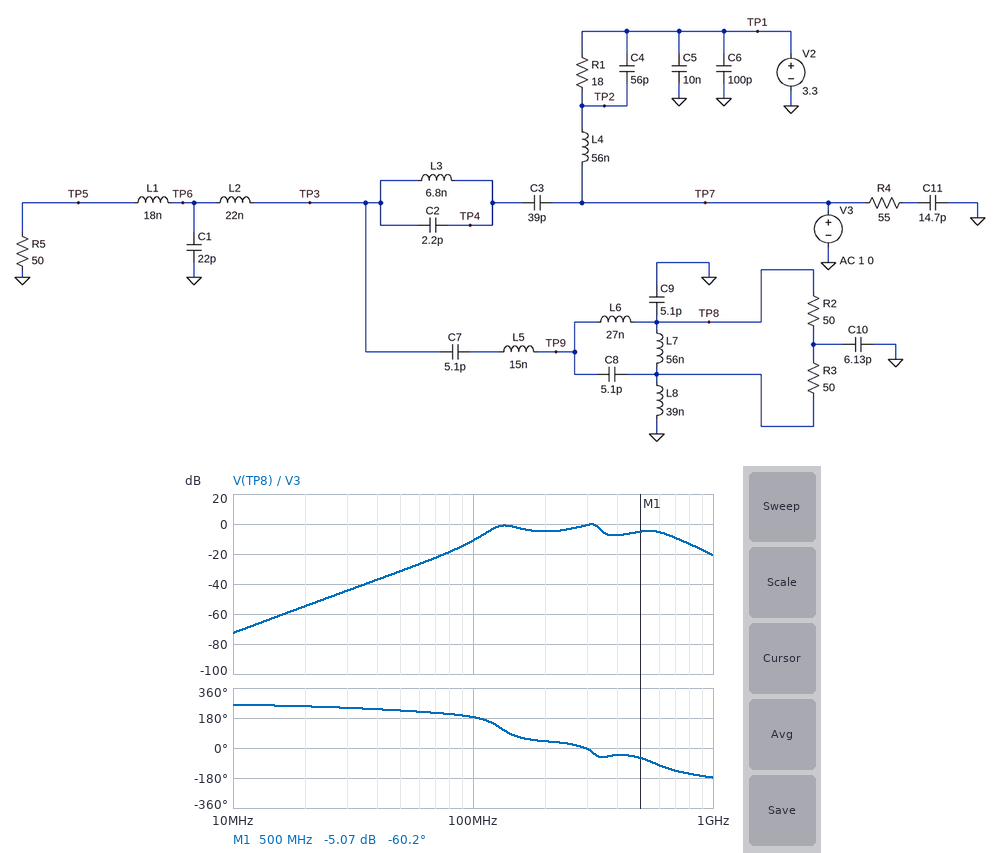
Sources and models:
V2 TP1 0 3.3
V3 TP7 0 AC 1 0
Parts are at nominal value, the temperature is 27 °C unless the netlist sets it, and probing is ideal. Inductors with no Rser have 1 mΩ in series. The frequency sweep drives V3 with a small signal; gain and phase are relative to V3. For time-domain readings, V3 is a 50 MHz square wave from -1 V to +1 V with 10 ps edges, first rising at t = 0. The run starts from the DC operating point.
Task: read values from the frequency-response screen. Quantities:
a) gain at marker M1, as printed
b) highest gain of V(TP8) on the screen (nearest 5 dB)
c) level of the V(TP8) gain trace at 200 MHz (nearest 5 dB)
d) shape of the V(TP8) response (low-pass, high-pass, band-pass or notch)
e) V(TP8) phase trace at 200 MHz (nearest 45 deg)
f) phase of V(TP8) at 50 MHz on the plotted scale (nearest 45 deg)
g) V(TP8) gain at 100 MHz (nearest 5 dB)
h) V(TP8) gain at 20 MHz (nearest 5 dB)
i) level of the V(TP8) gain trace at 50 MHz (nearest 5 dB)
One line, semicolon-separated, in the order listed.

-5.07 dB; 0 dB; -5 dB; band-pass; 45 deg; 225 deg; -10 dB; -55 dB; -30 dB
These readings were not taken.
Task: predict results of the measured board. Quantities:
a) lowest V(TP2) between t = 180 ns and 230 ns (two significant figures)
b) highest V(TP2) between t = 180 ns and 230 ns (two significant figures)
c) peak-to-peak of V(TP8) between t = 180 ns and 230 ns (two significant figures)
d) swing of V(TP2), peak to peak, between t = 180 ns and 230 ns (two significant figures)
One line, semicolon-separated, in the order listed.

-1.0 V; 1.0 V; 1.5 V; 2.0 V
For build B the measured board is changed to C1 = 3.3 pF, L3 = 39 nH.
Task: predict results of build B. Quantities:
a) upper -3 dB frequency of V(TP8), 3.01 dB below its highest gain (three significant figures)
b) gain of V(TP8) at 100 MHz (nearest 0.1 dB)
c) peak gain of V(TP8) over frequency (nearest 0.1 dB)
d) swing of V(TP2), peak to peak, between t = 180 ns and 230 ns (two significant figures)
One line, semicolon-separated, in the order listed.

151 MHz; -7.1 dB; 2.2 dB; 2.0 V
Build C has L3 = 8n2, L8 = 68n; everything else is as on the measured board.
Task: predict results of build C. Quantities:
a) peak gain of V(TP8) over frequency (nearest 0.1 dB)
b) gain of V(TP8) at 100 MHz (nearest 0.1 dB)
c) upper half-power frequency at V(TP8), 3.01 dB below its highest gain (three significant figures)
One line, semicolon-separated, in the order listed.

1.8 dB; -5.2 dB; 135 MHz
